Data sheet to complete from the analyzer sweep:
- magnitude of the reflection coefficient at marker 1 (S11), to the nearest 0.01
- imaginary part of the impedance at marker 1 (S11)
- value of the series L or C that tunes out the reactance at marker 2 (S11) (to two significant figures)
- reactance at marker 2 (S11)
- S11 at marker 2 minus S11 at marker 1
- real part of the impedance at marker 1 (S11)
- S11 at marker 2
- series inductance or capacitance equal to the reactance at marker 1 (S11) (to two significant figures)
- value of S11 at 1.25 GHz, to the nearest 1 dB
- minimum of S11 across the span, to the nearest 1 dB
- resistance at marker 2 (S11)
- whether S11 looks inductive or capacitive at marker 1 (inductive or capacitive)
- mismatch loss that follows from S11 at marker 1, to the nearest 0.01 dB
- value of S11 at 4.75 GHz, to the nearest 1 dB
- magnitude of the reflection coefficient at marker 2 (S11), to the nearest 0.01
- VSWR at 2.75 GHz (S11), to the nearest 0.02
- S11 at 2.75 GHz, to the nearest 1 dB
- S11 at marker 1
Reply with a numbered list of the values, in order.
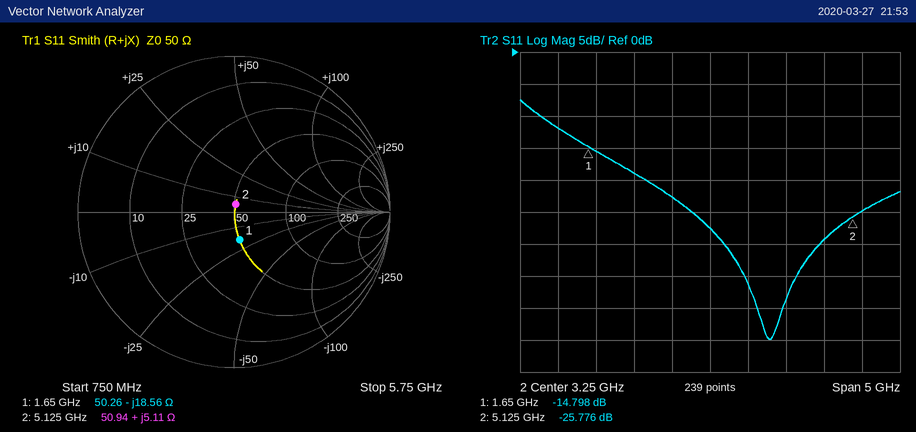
1. 0.18
2. -18.56 Ω
3. 6.1 pF
4. +5.11 Ω
5. -10.978 dB
6. 50.26 Ω
7. -25.776 dB
8. 5.2 pF
9. -12 dB
10. -45 dB
11. 50.94 Ω
12. capacitive
13. 0.15 dB
14. -29 dB
15. 0.05
16. 1.16
17. -23 dB
18. -14.798 dB
